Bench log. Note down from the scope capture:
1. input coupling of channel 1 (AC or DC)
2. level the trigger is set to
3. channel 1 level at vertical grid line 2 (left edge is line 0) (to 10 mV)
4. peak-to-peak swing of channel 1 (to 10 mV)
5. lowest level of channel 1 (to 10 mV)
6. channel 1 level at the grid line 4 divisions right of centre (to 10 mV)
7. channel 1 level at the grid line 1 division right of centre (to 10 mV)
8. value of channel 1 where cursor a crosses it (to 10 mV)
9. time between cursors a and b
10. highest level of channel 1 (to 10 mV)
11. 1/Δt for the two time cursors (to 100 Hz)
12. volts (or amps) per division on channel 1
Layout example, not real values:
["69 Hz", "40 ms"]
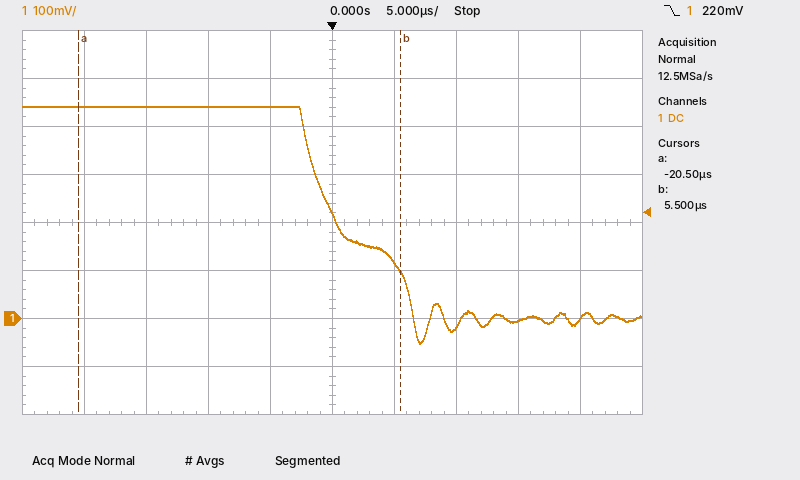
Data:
["DC", "220 mV", "440 mV", "490 mV", "-50 mV", "0 mV", "120 mV", "440 mV", "26.0 µs", "440 mV", "38.5 kHz", "100 mV"]
